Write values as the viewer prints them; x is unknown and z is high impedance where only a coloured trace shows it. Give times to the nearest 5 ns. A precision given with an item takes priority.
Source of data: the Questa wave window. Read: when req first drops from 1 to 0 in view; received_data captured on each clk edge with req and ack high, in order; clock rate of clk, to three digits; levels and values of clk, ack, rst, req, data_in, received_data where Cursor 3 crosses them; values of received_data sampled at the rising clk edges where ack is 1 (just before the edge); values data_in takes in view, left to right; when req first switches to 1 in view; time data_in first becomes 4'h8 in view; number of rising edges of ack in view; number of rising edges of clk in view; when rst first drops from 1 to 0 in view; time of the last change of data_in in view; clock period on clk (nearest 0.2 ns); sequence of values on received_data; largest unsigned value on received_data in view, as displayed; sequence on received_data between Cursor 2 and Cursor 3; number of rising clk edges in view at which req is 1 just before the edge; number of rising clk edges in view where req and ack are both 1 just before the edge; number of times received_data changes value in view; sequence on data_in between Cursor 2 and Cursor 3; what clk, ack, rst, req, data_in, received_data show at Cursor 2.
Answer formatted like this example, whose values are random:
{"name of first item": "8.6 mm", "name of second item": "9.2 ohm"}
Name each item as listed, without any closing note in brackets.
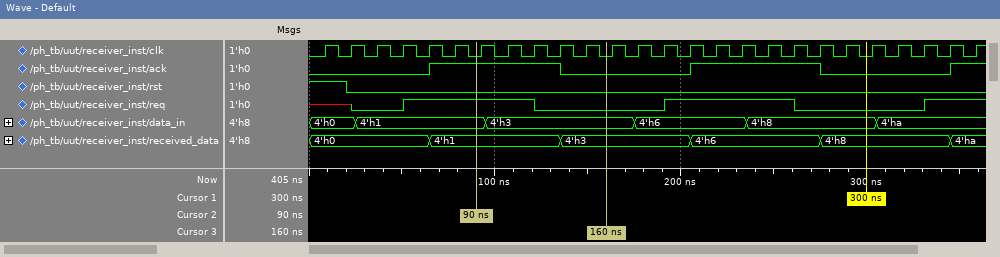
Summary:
{"when req first drops from 1 to 0 in view": "120 ns", "received_data captured on each clk edge with req and ack high, in order": "4'h1, 4'h1, 4'h1, 4'h1, 4'h6, 4'h6, 4'h6, 4'h6, 4'ha", "clock rate of clk, to three digits": "71.4 MHz", "levels and values of clk, ack, rst, req, data_in, received_data where Cursor 3 crosses them": "clk=0, ack=0, rst=0, req=0, data_in=4'h3, received_data=4'h3", "values of received_data sampled at the rising clk edges where ack is 1": "4'h1, 4'h1, 4'h1, 4'h1, 4'h1, 4'h6, 4'h6, 4'h6, 4'h6, 4'h6, 4'ha", "values data_in takes in view, left to right": "4'h0, 4'h1, 4'h3, 4'h6, 4'h8, 4'ha", "when req first switches to 1 in view": "50 ns", "time data_in first becomes 4'h8 in view": "235 ns", "number of rising edges of ack in view": "3", "number of rising edges of clk in view": "26", "when rst first drops from 1 to 0 in view": "20 ns", "time of the last change of data_in in view": "305 ns", "clock period on clk": "14 ns", "sequence of values on received_data": "4'h0, 4'h1, 4'h3, 4'h6, 4'h8, 4'ha", "largest unsigned value on received_data in view, as displayed": "4'ha", "sequence on received_data between Cursor 2 and Cursor 3": "4'h1, 4'h3", "number of rising clk edges in view at which req is 1 just before the edge": "12", "number of rising clk edges in view where req and ack are both 1 just before the edge": "9", "number of times received_data changes value in view": "5", "sequence on data_in between Cursor 2 and Cursor 3": "4'h1, 4'h3", "what clk, ack, rst, req, data_in, received_data show at Cursor 2": "clk=0, ack=1, rst=0, req=1, data_in=4'h1, received_data=4'h1"}
